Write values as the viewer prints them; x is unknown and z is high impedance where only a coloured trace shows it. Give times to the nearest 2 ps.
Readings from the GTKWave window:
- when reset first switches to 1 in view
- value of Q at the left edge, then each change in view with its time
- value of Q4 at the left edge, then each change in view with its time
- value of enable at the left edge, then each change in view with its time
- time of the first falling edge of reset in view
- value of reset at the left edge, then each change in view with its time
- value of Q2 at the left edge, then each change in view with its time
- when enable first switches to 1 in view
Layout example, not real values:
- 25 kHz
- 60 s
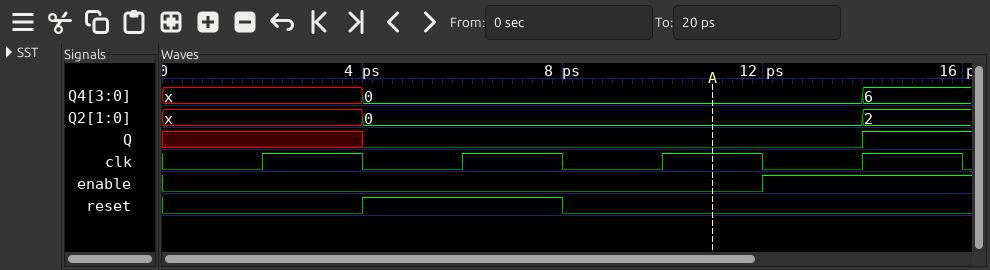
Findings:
- 4 ps
- x, 0 at 4 ps, 1 at 14 ps
- x, 0 at 4 ps, 6 at 14 ps
- 0, 1 at 12 ps
- 8 ps
- 0, 1 at 4 ps, 0 at 8 ps
- x, 0 at 4 ps, 2 at 14 ps
- 12 ps
